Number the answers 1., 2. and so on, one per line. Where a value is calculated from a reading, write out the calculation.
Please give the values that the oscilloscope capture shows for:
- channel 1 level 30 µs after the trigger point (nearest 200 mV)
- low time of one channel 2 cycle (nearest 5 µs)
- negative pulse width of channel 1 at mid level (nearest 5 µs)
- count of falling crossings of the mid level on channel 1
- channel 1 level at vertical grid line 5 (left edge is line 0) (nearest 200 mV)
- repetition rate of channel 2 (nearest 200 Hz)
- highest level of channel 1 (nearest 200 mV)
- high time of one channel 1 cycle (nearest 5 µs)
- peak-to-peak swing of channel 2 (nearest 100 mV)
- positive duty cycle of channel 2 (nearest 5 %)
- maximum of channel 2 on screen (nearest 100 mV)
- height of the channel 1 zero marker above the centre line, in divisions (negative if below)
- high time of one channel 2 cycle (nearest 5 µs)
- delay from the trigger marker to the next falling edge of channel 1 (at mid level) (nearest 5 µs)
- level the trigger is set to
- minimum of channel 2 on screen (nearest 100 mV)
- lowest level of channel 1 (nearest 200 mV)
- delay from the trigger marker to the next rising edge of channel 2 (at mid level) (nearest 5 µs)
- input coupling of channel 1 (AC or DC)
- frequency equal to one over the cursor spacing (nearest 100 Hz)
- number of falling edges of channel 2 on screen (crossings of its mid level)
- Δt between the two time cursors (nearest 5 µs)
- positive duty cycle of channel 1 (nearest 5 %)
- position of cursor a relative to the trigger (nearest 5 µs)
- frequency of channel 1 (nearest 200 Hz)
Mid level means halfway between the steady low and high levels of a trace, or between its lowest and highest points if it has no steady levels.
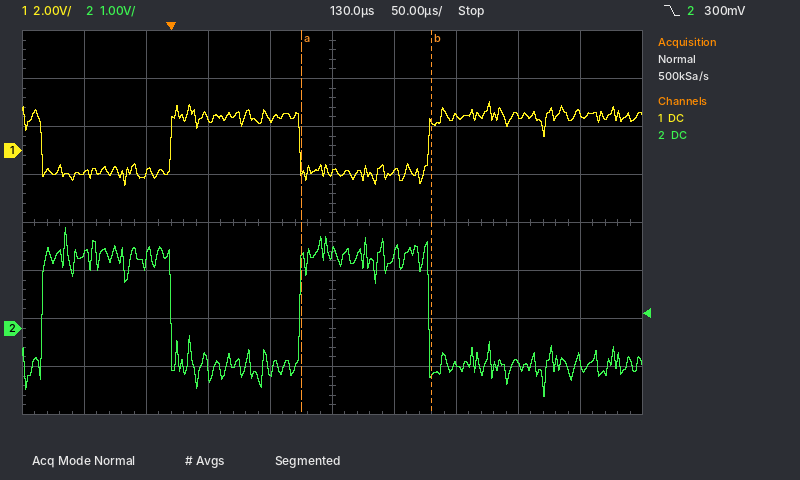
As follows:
1. 1.4 V
2. 105 µs
3. 105 µs
4. 2
5. -1.0 V
6. 4.8 kHz
7. 2.0 V
8. 105 µs
9. 2.1 V − (-1.4 V) = 3.5 V
10. 50 %
11. 2.1 V
12. +1.5 div
13. 105 µs
14. 105 µs
15. 300 mV
16. -1.4 V
17. -1.4 V
18. 105 µs
19. DC
20. 1 / 105 µs ≈ 9.5 kHz
21. 2
22. 105 µs
23. 50 %
24. +105 µs
25. 4.8 kHz
